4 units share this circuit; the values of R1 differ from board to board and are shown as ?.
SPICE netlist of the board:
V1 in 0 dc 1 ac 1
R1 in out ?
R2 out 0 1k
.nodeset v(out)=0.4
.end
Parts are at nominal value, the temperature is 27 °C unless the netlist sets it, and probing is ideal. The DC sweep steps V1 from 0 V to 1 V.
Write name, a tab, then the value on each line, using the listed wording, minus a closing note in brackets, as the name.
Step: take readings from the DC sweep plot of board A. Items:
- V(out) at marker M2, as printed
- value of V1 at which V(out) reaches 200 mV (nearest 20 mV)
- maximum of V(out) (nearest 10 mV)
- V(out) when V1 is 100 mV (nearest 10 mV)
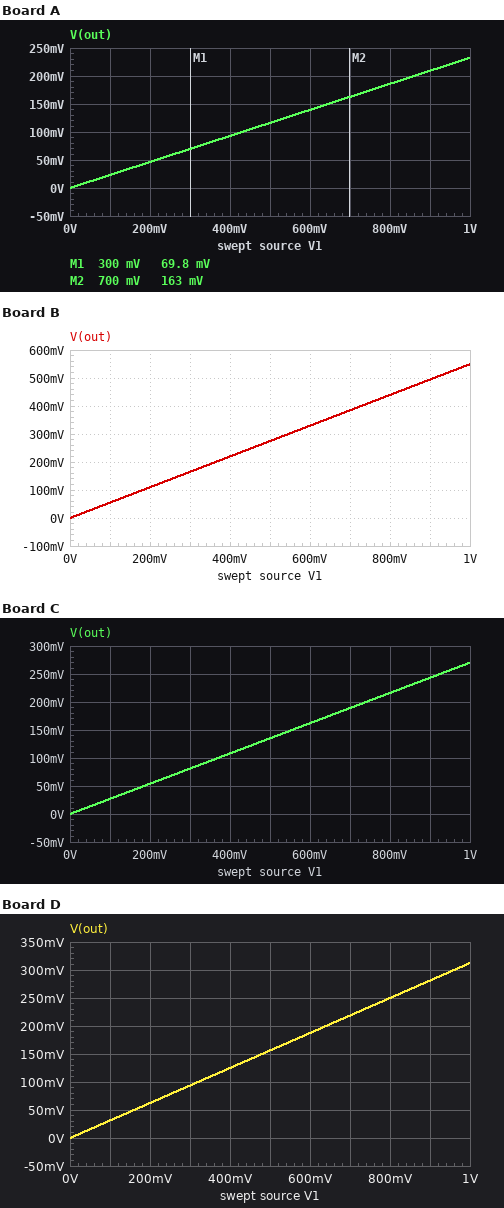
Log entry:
V(out) at marker M2, as printed	163 mV
value of V1 at which V(out) reaches 200 mV	860 mV
maximum of V(out)	230 mV
V(out) when V1 is 100 mV	20 mV
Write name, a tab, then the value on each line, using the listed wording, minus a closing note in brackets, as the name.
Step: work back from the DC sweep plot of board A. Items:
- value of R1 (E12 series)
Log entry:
value of R1	3.3 kΩ
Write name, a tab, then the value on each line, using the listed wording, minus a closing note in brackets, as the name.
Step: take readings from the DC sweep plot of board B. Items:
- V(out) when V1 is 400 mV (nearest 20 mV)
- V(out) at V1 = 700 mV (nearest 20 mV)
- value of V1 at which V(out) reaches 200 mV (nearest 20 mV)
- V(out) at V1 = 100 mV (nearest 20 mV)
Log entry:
V(out) when V1 is 400 mV	220 mV
V(out) at V1 = 700 mV	380 mV
value of V1 at which V(out) reaches 200 mV	360 mV
V(out) at V1 = 100 mV	60 mV
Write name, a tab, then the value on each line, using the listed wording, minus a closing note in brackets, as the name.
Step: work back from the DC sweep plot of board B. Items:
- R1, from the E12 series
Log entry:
R1, from the E12 series	820 Ω
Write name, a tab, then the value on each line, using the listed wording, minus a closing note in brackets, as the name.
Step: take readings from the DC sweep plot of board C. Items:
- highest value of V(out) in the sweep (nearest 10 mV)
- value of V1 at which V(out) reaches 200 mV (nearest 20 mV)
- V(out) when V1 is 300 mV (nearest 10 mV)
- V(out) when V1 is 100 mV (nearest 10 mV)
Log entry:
highest value of V(out) in the sweep	270 mV
value of V1 at which V(out) reaches 200 mV	740 mV
V(out) when V1 is 300 mV	80 mV
V(out) when V1 is 100 mV	30 mV
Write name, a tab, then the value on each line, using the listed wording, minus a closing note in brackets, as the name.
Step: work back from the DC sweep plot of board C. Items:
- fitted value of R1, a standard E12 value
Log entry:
fitted value of R1, a standard E12 value	2.7 kΩ
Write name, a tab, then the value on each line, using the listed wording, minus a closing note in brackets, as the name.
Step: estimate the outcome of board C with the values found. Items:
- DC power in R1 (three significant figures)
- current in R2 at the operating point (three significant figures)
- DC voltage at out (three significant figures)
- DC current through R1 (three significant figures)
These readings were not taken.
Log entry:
DC power in R1	197 µW
current in R2 at the operating point	270 µA
DC voltage at out	270 mV
DC current through R1	270 µA
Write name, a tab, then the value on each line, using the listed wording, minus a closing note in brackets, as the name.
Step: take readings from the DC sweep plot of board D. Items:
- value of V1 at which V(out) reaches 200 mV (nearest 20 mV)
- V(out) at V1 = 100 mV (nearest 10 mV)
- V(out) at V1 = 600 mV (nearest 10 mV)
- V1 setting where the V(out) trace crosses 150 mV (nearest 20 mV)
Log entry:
value of V1 at which V(out) reaches 200 mV	640 mV
V(out) at V1 = 100 mV	30 mV
V(out) at V1 = 600 mV	190 mV
V1 setting where the V(out) trace crosses 150 mV	480 mV
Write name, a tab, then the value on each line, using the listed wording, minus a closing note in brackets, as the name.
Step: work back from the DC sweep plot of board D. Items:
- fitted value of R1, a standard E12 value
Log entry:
fitted value of R1, a standard E12 value	2.2 kΩ
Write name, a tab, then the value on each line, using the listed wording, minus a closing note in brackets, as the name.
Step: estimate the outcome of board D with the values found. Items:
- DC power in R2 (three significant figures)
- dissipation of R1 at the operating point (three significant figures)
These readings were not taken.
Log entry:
DC power in R2	97.7 µW
dissipation of R1 at the operating point	215 µW
